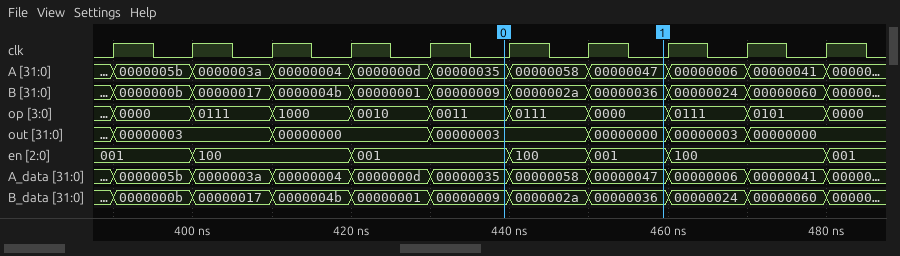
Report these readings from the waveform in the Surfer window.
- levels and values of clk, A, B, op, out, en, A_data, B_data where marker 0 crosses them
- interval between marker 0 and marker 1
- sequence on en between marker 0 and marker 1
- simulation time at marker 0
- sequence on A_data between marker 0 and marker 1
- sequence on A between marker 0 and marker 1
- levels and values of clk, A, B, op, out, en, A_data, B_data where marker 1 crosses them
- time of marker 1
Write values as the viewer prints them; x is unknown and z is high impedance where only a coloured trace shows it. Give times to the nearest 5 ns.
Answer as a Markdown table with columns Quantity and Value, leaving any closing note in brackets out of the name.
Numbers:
| Quantity | Value |
|---|---|
| levels and values of clk, A, B, op, out, en, A_data, B_data where marker 0 crosses them | clk=0, A=00000035, B=00000009, op=0011, out=00000003, en=001, A_data=00000035, B_data=00000009 |
| interval between marker 0 and marker 1 | 20 ns |
| sequence on en between marker 0 and marker 1 | 001, 100, 001 |
| simulation time at marker 0 | 440 ns |
| sequence on A_data between marker 0 and marker 1 | 00000035, 00000058, 00000047 |
| sequence on A between marker 0 and marker 1 | 00000035, 00000058, 00000047 |
| levels and values of clk, A, B, op, out, en, A_data, B_data where marker 1 crosses them | clk=0, A=00000047, B=00000036, op=0000, out=00000000, en=001, A_data=00000047, B_data=00000036 |
| time of marker 1 | 460 ns |
